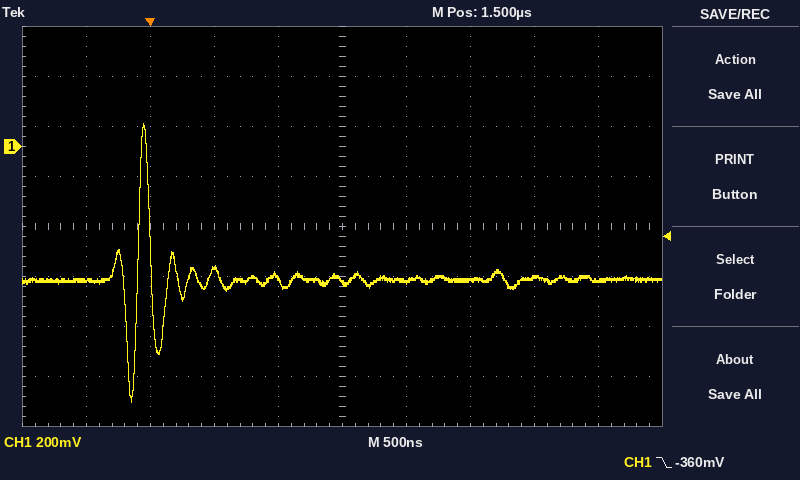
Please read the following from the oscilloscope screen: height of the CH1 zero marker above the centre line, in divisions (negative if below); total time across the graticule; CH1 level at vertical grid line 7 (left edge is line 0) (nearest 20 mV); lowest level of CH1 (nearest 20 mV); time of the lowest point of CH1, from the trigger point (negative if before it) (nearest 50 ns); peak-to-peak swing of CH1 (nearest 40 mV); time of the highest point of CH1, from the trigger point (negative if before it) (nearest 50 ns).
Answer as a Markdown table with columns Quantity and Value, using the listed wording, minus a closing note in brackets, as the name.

| Quantity | Value |
|---|---|
| height of the CH1 zero marker above the centre line, in divisions | +1.6 div |
| total time across the graticule | 5 µs |
| CH1 level at vertical grid line 7 (left edge is line 0) | -540 mV |
| lowest level of CH1 | -1.02 V |
| time of the lowest point of CH1, from the trigger point (negative if before it) | -150 ns |
| peak-to-peak swing of CH1 | 1.12 V |
| time of the highest point of CH1, from the trigger point (negative if before it) | -50 ns |
